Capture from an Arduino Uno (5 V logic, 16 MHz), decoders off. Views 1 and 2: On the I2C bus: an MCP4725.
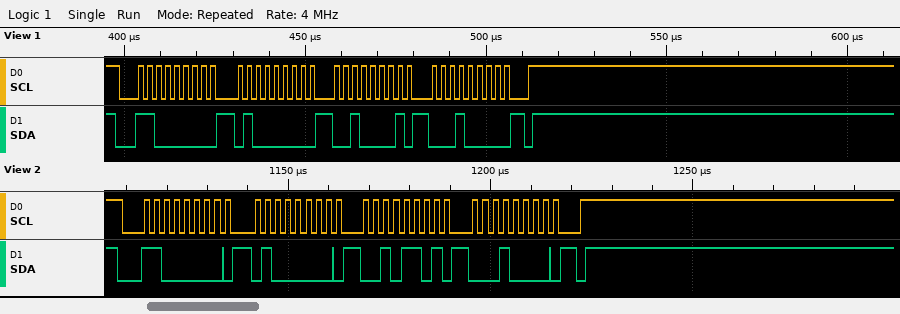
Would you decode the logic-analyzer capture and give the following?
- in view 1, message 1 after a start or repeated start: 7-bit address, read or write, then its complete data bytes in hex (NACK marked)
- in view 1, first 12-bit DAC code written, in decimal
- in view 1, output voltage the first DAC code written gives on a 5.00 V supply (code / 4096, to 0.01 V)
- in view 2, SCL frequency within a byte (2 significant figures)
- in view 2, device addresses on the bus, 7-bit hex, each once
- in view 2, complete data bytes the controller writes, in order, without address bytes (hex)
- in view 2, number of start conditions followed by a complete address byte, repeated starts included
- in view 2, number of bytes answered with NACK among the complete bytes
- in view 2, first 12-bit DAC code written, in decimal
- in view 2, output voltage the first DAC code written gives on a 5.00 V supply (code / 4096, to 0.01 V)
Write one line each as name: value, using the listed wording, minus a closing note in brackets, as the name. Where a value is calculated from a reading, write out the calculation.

in view 1, message 1 after a start or repeated start: 7-bit address, read or write, then its complete data bytes in hex: 0x60 write: 40 21 10
in view 1, first 12-bit DAC code written, in decimal: 529
in view 1, output voltage the first DAC code written gives on a 5.00 V supply: 529 / 4096 x 5.00 V = 0.65 V
in view 2, SCL frequency within a byte: 400 kHz
in view 2, device addresses on the bus, 7-bit hex, each once: 0x60
in view 2, complete data bytes the controller writes, in order, without address bytes: 40 2D 10
in view 2, number of start conditions followed by a complete address byte, repeated starts included: 1
in view 2, number of bytes answered with NACK among the complete bytes: 0
in view 2, first 12-bit DAC code written, in decimal: 721
in view 2, output voltage the first DAC code written gives on a 5.00 V supply: 721 / 4096 x 5.00 V = 0.88 V
